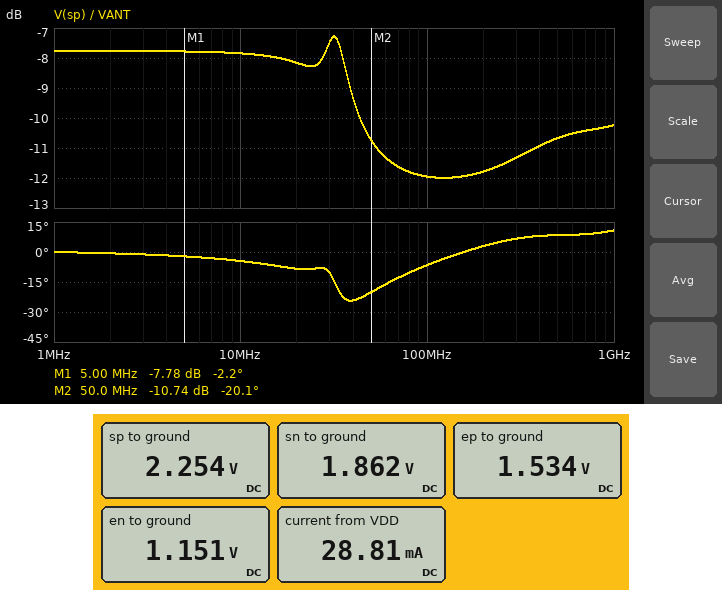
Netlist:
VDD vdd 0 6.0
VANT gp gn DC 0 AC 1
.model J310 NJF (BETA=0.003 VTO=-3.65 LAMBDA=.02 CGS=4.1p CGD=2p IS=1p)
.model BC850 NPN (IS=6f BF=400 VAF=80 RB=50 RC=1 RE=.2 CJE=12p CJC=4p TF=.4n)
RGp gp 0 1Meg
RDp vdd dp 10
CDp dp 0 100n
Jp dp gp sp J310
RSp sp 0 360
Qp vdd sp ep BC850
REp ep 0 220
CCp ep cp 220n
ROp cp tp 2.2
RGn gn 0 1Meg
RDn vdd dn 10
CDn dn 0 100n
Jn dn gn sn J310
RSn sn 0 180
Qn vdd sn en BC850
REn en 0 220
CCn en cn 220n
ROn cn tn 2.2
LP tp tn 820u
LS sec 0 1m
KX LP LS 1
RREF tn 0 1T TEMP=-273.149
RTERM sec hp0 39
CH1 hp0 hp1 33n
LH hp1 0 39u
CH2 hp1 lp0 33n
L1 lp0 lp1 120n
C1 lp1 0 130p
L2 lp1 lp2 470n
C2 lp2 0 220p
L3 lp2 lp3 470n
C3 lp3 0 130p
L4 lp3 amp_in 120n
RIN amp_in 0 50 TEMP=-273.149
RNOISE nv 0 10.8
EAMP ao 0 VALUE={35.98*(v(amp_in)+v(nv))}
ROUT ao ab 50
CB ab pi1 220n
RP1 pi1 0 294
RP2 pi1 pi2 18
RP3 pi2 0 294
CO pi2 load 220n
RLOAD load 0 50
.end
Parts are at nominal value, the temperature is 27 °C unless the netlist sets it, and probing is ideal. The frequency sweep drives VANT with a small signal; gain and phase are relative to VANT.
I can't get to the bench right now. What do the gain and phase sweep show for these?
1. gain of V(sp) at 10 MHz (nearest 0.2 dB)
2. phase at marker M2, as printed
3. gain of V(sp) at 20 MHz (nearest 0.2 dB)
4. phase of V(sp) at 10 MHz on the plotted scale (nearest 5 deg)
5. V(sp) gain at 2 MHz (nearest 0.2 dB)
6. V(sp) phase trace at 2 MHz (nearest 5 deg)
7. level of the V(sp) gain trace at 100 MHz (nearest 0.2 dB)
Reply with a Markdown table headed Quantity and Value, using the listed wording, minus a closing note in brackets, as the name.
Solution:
| Quantity | Value |
|---|---|
| gain of V(sp) at 10 MHz | -7.8 dB |
| phase at marker M2, as printed | -20.1 deg |
| gain of V(sp) at 20 MHz | -8.2 dB |
| phase of V(sp) at 10 MHz on the plotted scale | -5 deg |
| V(sp) gain at 2 MHz | -7.8 dB |
| V(sp) phase trace at 2 MHz | 0 deg |
| level of the V(sp) gain trace at 100 MHz | -12.0 dB |
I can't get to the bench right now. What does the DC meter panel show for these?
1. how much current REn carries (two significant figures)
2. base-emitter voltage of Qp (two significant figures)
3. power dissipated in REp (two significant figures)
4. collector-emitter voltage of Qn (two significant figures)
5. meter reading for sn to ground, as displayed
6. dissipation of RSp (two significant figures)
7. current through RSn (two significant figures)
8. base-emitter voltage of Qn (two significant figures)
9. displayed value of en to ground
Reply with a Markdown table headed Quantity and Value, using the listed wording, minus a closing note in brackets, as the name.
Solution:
| Quantity | Value |
|---|---|
| how much current REn carries | 5.2 mA |
| base-emitter voltage of Qp | 720 mV |
| power dissipated in REp | 11 mW |
| collector-emitter voltage of Qn | 4.8 V |
| meter reading for sn to ground, as displayed | 1.862 V |
| dissipation of RSp | 14 mW |
| current through RSn | 10 mA |
| base-emitter voltage of Qn | 710 mV |
| displayed value of en to ground | 1.151 V |
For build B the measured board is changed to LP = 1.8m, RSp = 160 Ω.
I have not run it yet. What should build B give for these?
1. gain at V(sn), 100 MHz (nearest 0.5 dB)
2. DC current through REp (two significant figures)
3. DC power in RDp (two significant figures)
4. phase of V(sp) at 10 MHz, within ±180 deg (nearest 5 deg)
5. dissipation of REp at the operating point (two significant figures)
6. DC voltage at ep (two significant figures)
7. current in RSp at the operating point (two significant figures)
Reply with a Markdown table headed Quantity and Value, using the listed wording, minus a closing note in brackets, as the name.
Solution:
| Quantity | Value |
|---|---|
| gain at V(sn), 100 MHz | -11.5 dB |
| DC current through REp | 4.9 mA |
| DC power in RDp | 1.3 mW |
| phase of V(sp) at 10 MHz, within ±180 deg | 0 deg |
| dissipation of REp at the operating point | 5.3 mW |
| DC voltage at ep | 1.1 V |
| current in RSp at the operating point | 11 mA |
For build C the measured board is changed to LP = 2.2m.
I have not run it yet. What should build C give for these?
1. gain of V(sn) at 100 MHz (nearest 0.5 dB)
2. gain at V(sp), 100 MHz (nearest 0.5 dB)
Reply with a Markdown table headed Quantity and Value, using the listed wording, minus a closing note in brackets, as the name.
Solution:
| Quantity | Value |
|---|---|
| gain of V(sn) at 100 MHz | -11.5 dB |
| gain at V(sp), 100 MHz | -10.5 dB |
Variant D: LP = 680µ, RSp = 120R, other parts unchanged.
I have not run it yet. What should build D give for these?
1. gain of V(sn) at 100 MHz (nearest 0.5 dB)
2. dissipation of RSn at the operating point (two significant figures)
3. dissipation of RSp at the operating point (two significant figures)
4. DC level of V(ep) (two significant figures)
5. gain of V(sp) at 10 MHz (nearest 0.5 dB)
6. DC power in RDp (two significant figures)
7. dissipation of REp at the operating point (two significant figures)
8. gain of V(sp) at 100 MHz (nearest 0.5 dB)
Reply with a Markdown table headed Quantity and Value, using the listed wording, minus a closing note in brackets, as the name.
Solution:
| Quantity | Value |
|---|---|
| gain of V(sn) at 100 MHz | -12.0 dB |
| dissipation of RSn at the operating point | 19 mW |
| dissipation of RSp at the operating point | 22 mW |
| DC level of V(ep) | 910 mV |
| gain of V(sp) at 10 MHz | -11.0 dB |
| DC power in RDp | 1.8 mW |
| dissipation of REp at the operating point | 3.8 mW |
| gain of V(sp) at 100 MHz | -13.5 dB |
